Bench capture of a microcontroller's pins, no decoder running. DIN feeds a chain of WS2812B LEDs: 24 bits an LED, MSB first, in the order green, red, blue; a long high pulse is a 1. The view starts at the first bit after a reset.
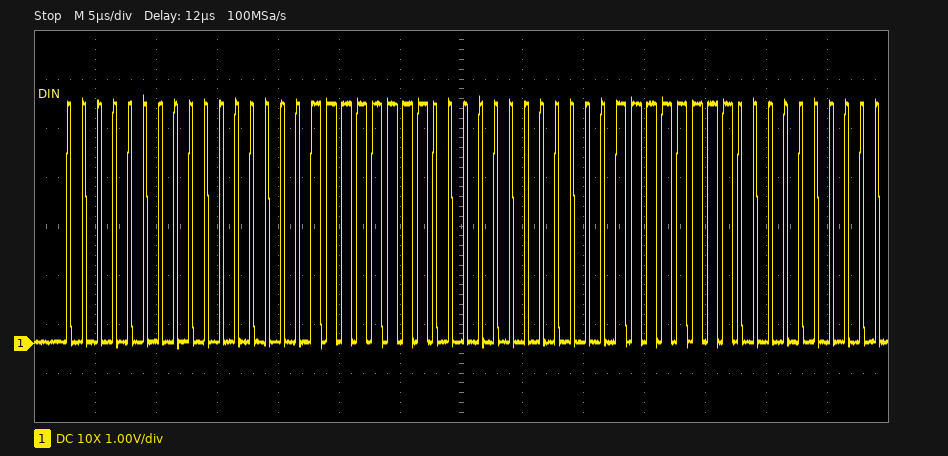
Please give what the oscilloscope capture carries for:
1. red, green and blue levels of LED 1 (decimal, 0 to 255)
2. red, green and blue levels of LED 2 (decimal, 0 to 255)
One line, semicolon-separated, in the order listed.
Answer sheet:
0, 0, 255; 15, 0, 240
